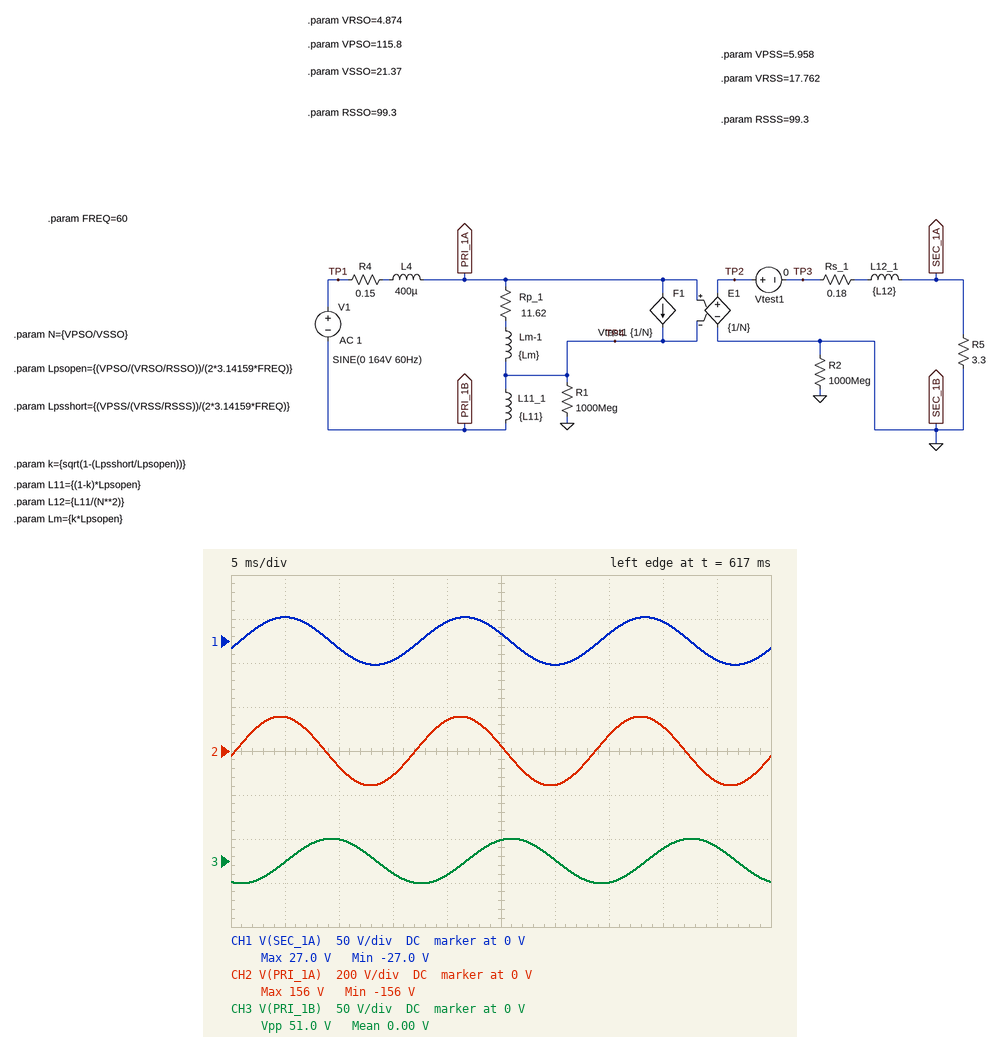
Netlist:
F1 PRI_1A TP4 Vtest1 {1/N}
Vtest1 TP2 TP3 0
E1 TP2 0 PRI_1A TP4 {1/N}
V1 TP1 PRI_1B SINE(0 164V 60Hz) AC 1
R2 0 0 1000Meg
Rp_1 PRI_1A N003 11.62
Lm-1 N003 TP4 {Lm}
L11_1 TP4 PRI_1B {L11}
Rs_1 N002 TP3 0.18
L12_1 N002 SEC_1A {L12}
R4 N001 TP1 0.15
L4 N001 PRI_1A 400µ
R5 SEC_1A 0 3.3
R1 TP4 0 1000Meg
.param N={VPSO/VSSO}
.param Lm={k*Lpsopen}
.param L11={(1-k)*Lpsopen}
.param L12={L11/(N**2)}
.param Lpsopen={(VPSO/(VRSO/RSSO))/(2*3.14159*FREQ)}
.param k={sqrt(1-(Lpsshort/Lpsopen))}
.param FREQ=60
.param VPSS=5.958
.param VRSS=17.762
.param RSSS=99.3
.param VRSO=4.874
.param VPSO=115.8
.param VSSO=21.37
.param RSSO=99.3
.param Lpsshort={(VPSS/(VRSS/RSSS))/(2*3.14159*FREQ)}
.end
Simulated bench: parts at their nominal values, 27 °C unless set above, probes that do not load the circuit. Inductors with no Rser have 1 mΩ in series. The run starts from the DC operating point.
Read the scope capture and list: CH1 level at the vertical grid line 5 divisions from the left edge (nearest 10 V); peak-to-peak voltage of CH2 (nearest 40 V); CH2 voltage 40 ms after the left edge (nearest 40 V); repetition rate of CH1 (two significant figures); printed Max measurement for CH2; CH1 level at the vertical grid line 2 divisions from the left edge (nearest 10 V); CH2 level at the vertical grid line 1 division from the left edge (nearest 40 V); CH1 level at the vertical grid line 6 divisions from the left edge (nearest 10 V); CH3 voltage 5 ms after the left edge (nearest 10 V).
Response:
10 V
320 V
120 V
60 Hz
156 V
-10 V
160 V
-30 V
0 V
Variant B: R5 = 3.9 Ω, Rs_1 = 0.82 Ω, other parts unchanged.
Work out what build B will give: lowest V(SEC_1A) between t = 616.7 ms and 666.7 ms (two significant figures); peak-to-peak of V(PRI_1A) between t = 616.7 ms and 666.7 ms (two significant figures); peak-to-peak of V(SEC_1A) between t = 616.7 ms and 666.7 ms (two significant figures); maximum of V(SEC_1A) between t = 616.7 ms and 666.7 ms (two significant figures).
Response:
-24 V
320 V
48 V
24 V
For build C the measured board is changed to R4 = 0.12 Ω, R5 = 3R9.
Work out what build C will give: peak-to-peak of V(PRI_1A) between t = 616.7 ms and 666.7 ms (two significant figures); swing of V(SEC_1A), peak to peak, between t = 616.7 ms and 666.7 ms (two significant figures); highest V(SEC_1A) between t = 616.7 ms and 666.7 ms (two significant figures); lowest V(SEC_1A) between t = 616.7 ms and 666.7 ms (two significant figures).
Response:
320 V
55 V
28 V
-28 V
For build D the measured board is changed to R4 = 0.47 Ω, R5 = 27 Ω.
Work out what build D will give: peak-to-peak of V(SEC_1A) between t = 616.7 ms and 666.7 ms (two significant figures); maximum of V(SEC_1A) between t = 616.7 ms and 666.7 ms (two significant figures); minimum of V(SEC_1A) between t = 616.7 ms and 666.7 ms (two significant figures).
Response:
60 V
30 V
-30 V
